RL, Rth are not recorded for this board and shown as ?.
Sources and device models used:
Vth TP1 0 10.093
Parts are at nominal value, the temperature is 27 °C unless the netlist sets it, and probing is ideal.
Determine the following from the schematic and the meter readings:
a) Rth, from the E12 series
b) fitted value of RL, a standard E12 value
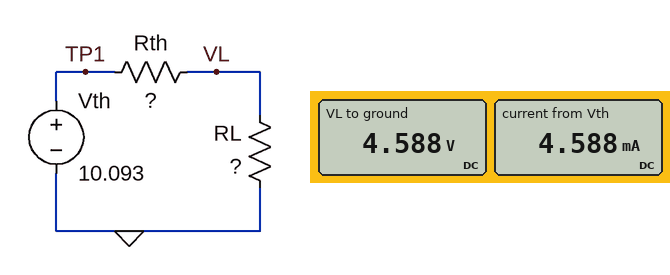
1.2 kΩ
1 kΩ
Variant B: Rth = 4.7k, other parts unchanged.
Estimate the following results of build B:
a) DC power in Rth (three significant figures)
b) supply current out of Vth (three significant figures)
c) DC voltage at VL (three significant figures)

14.7 mW
1.77 mA
1.77 V
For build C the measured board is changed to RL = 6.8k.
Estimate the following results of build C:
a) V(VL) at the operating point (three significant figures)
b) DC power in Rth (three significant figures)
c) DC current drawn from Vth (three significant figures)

8.58 V
1.91 mW
1.26 mA
